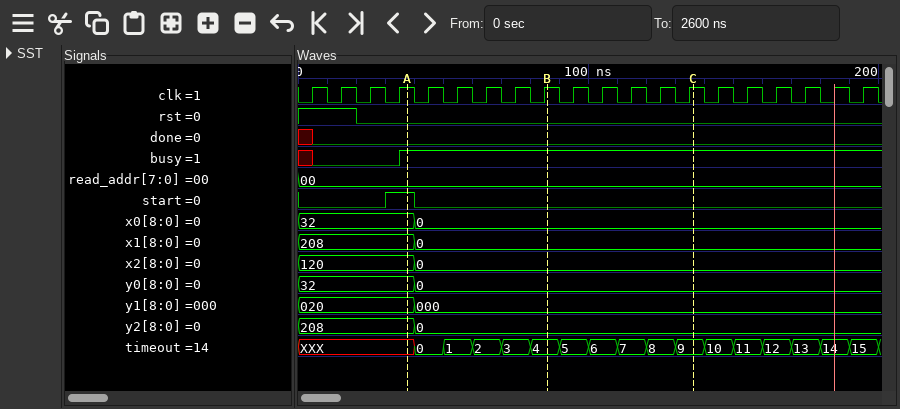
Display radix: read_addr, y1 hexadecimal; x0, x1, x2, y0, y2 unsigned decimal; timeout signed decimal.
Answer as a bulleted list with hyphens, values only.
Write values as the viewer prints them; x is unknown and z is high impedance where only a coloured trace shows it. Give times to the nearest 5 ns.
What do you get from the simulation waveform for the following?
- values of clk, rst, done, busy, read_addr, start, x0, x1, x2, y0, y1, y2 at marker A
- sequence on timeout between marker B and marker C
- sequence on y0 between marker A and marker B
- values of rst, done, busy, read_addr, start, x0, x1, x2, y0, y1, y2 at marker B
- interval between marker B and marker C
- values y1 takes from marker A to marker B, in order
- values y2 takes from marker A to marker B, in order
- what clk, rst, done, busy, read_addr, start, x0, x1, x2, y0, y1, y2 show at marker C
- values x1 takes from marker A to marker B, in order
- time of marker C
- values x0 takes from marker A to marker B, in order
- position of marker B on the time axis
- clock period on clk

- clk=1, rst=0, done=0, busy=1, read_addr=00, start=1, x0=32, x1=208, x2=120, y0=32, y1=020, y2=208
- 4, 5, 6, 7, 8, 9
- 32, 0
- rst=0, done=0, busy=1, read_addr=00, start=0, x0=0, x1=0, x2=0, y0=0, y1=000, y2=0
- 50 ns
- 020, 000
- 208, 0
- clk=1, rst=0, done=0, busy=1, read_addr=00, start=0, x0=0, x1=0, x2=0, y0=0, y1=000, y2=0
- 208, 0
- 135 ns
- 32, 0
- 85 ns
- 10 ns
